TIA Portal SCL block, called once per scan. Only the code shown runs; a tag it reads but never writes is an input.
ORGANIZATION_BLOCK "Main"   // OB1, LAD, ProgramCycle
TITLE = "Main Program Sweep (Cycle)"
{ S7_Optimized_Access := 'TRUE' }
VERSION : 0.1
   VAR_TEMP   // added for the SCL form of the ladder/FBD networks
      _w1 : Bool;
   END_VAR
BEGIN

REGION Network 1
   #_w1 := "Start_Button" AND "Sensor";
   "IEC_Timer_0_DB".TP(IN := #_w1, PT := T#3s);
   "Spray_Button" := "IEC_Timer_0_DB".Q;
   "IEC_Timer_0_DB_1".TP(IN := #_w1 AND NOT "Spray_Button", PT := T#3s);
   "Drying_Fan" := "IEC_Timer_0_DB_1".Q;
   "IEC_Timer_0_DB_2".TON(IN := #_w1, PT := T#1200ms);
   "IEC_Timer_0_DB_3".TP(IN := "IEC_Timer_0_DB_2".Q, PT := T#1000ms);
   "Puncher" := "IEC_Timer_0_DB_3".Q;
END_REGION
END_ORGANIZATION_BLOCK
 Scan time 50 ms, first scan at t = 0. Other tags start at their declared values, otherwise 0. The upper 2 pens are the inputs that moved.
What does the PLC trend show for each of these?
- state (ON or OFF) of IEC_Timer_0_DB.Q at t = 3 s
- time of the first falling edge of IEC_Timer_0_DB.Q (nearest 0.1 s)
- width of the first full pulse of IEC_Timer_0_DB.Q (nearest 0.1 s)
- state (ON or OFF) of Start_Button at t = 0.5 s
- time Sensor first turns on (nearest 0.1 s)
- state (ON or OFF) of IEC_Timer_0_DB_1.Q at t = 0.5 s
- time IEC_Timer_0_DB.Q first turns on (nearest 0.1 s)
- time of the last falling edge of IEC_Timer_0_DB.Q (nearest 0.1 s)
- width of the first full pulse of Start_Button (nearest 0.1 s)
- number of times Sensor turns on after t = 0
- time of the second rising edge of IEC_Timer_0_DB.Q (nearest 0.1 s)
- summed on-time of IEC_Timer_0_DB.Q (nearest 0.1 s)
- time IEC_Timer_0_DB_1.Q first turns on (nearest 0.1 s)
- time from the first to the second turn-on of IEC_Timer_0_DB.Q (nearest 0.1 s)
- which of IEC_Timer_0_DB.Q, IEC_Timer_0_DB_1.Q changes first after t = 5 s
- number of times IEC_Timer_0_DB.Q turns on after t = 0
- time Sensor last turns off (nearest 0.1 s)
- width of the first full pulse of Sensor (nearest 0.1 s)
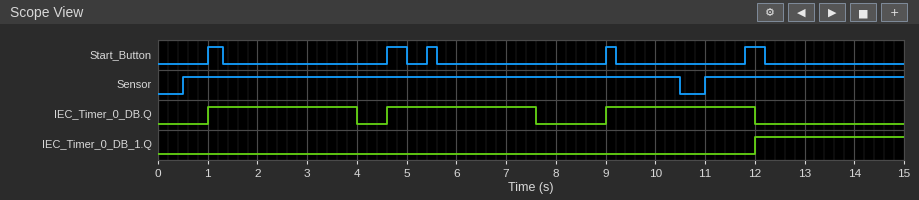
ON
4.0 s
3.0 s
OFF
0.5 s
OFF
1.0 s
12.0 s
0.3 s
2
4.6 s
9.0 s
12.0 s
3.6 s
IEC_Timer_0_DB.Q
3
10.5 s
10.0 s
